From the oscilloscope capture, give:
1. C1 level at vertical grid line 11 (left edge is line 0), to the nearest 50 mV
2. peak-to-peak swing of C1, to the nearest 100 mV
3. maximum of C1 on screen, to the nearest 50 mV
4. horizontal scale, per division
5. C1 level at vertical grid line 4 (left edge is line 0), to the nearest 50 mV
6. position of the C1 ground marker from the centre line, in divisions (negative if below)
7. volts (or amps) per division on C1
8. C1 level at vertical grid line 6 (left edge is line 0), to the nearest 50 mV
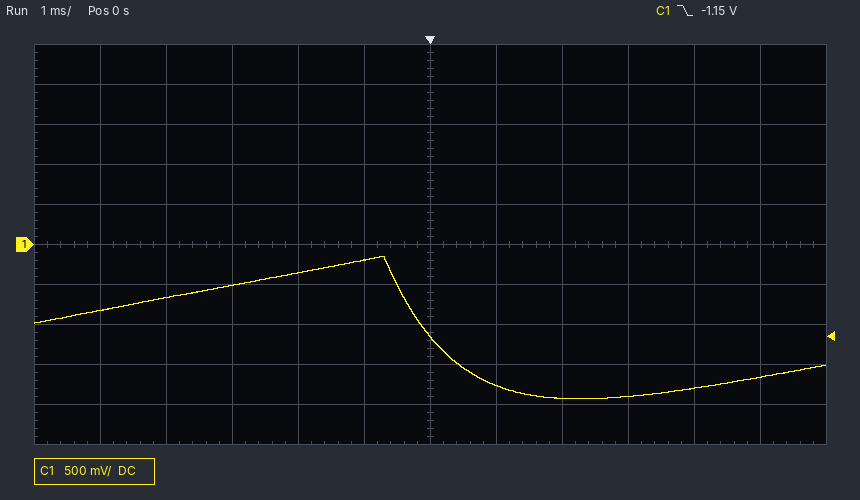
-1.65 V
1.80 V
-150 mV
1 ms
-350 mV
0.0 div
500 mV
-1.15 V
